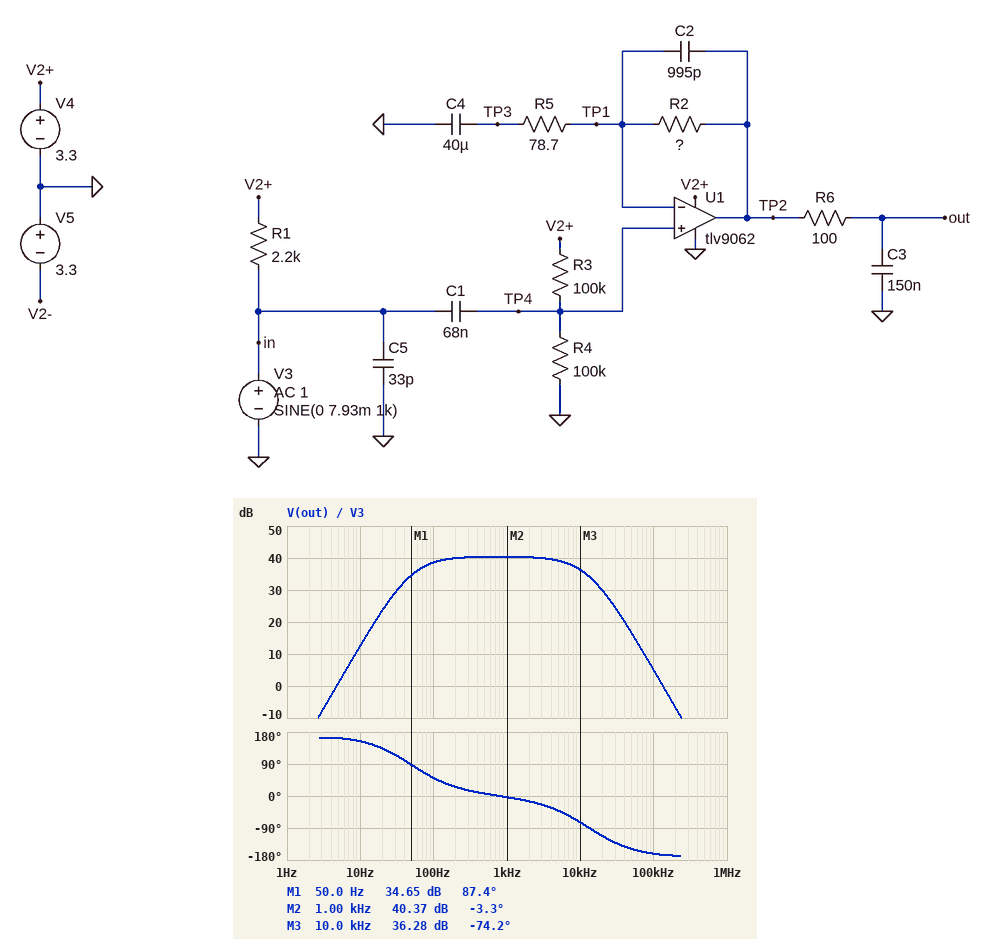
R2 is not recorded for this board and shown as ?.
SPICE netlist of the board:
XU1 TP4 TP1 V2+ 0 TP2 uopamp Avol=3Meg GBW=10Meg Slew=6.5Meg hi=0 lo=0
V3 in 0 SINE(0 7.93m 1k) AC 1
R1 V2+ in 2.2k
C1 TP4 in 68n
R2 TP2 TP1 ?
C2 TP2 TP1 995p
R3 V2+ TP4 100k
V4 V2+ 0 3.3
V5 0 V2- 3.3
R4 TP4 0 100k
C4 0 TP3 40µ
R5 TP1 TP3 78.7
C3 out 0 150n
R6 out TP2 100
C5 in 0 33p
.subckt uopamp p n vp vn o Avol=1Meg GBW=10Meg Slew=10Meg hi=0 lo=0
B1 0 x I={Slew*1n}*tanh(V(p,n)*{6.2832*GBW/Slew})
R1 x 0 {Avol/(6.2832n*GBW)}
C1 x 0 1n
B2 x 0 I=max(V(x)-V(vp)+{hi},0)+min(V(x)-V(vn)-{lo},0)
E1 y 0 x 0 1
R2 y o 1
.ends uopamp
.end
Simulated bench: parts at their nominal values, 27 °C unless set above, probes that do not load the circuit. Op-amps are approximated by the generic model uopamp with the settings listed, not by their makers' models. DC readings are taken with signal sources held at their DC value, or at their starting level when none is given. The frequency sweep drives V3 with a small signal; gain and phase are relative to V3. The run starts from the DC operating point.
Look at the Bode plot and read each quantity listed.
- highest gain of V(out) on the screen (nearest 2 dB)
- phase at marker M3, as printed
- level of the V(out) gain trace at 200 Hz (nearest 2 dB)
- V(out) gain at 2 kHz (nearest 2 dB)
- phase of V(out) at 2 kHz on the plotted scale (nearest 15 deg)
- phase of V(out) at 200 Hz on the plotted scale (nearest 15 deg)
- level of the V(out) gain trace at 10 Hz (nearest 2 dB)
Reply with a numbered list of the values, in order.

1. 40 dB
2. -74.2 deg
3. 40 dB
4. 40 dB
5. -15 deg
6. 30 deg
7. 12 dB
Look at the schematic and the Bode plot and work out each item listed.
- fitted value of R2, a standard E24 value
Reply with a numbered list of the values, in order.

1. 8.2 kΩ
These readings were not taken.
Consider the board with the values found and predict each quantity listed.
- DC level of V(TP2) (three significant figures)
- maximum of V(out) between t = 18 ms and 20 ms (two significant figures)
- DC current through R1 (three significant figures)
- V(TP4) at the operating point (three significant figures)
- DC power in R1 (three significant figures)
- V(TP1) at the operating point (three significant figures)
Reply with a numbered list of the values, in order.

1. 1.65 V
2. 2.5 V
3. 1.50 mA
4. 1.65 V
5. 4.95 mW
6. 1.65 V
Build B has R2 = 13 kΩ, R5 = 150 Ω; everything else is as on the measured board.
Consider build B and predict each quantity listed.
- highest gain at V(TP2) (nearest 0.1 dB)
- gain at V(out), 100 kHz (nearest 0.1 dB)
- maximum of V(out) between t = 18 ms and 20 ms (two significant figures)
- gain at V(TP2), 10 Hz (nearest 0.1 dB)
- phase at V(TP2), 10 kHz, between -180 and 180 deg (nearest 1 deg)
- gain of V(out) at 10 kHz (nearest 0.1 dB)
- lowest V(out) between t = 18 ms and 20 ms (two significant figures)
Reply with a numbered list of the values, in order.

1. 38.8 dB
2. 0.2 dB
3. 2.3 V
4. 16.2 dB
5. -41 deg
6. 33.5 dB
7. 960 mV
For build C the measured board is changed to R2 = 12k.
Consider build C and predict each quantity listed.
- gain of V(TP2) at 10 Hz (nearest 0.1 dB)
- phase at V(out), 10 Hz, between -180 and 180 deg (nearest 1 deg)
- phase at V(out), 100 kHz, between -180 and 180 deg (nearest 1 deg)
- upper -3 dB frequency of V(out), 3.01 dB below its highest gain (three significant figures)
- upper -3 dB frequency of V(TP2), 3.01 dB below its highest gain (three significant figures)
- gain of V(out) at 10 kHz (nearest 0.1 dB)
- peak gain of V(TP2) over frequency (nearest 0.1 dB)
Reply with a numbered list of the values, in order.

1. 15.9 dB
2. 155 deg
3. -165 deg
4. 7.08 kHz
5. 11.2 kHz
6. 38.4 dB
7. 43.7 dB
